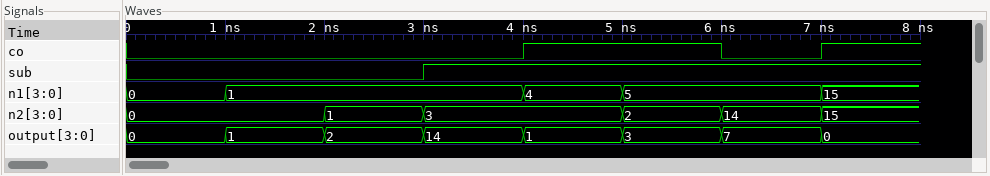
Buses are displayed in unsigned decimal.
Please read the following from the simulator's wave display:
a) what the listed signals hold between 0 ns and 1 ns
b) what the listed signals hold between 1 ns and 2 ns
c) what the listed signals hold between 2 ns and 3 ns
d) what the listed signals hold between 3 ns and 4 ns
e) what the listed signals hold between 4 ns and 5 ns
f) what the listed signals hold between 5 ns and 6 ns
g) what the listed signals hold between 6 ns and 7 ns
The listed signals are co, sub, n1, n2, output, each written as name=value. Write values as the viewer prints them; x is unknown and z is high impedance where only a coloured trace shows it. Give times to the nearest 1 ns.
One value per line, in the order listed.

co=0, sub=0, n1=0, n2=0, output=0
co=0, sub=0, n1=1, n2=0, output=1
co=0, sub=0, n1=1, n2=1, output=2
co=0, sub=1, n1=1, n2=3, output=14
co=1, sub=1, n1=4, n2=3, output=1
co=1, sub=1, n1=5, n2=2, output=3
co=0, sub=1, n1=5, n2=14, output=7
